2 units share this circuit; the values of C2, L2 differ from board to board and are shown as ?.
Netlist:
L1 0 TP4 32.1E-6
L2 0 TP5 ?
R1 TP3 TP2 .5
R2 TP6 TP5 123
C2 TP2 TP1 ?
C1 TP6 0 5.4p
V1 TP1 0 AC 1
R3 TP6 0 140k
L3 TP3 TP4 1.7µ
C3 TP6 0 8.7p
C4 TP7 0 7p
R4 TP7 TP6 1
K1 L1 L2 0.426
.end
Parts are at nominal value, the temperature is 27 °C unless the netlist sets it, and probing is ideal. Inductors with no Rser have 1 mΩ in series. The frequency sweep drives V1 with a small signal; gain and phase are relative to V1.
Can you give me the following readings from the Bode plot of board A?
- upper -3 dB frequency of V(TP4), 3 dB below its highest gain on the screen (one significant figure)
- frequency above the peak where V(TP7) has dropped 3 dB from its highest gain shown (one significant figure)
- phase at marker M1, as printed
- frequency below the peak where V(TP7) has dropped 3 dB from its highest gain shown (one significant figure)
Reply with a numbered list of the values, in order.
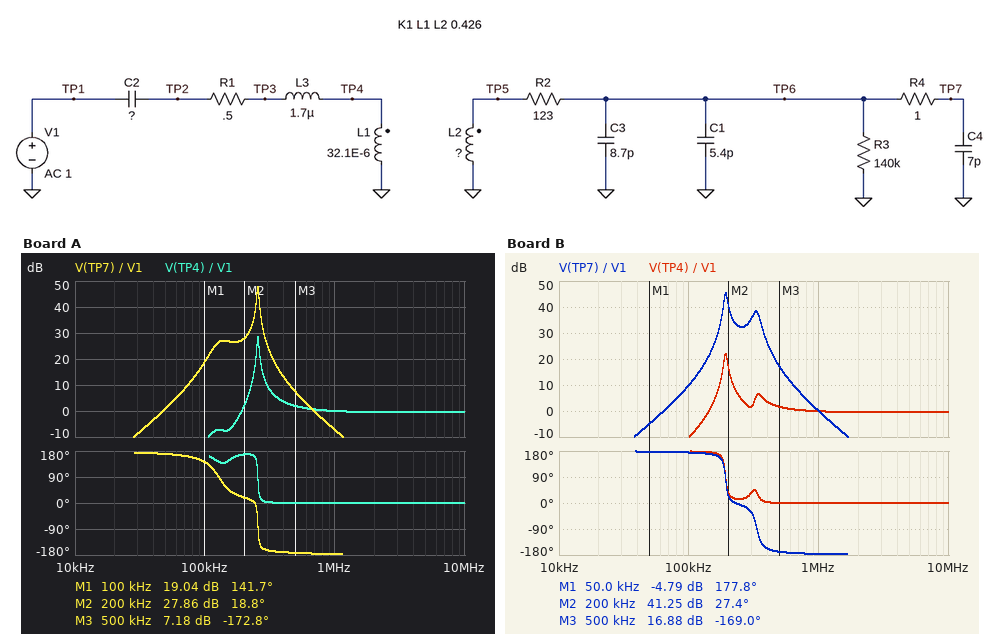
1. 300 kHz
2. 300 kHz
3. 141.7 deg
4. 300 kHz
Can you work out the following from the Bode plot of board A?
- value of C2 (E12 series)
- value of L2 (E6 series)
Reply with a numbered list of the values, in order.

1. 15 nF
2. 68 mH
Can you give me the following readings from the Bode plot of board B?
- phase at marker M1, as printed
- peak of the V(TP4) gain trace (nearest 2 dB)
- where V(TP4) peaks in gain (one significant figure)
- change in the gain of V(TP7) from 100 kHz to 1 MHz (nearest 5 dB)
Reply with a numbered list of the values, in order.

1. 177.8 deg
2. 22 dB
3. 200 kHz
4. -10 dB
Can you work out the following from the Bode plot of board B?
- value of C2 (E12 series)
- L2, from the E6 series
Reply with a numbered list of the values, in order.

1. 18 nF
2. 15 mH
